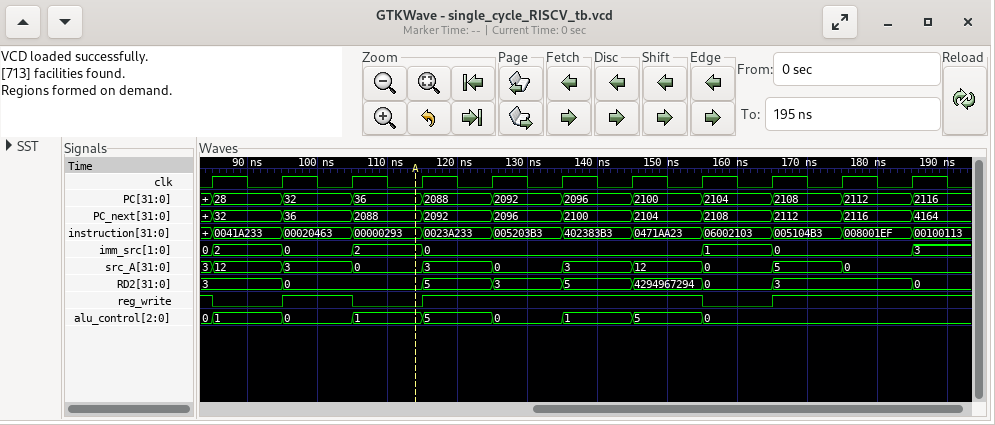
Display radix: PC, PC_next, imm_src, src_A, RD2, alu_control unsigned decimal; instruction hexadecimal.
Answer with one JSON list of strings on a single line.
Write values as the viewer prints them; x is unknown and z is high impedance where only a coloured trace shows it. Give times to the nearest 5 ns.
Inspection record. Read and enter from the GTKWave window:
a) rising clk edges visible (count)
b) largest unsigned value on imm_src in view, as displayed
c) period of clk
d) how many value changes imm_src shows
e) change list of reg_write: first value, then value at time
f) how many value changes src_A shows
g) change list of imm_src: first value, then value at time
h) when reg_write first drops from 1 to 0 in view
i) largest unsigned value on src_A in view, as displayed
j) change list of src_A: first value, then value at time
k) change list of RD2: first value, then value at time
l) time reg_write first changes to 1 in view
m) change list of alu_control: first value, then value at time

["11", "3", "10 ns", "7", "1, 0 at 85 ns, 1 at 95 ns, 0 at 105 ns, 1 at 115 ns, 0 at 155 ns, 1 at 165 ns", "10", "0, 2 at 85 ns, 0 at 95 ns, 2 at 105 ns, 0 at 115 ns, 1 at 155 ns, 0 at 165 ns, 3 at 185 ns", "85 ns", "12", "3, 12 at 85 ns, 3 at 95 ns, 0 at 105 ns, 3 at 115 ns, 0 at 125 ns, 3 at 135 ns, 12 at 145 ns, 0 at 155 ns, 5 at 165 ns, 0 at 175 ns", "3, 0 at 95 ns, 5 at 115 ns, 3 at 125 ns, 5 at 135 ns, 4294967294 at 145 ns, 0 at 155 ns, 3 at 165 ns, 0 at 185 ns", "95 ns", "0, 1 at 85 ns, 0 at 95 ns, 1 at 105 ns, 5 at 115 ns, 0 at 125 ns, 1 at 135 ns, 5 at 145 ns, 0 at 155 ns"]
